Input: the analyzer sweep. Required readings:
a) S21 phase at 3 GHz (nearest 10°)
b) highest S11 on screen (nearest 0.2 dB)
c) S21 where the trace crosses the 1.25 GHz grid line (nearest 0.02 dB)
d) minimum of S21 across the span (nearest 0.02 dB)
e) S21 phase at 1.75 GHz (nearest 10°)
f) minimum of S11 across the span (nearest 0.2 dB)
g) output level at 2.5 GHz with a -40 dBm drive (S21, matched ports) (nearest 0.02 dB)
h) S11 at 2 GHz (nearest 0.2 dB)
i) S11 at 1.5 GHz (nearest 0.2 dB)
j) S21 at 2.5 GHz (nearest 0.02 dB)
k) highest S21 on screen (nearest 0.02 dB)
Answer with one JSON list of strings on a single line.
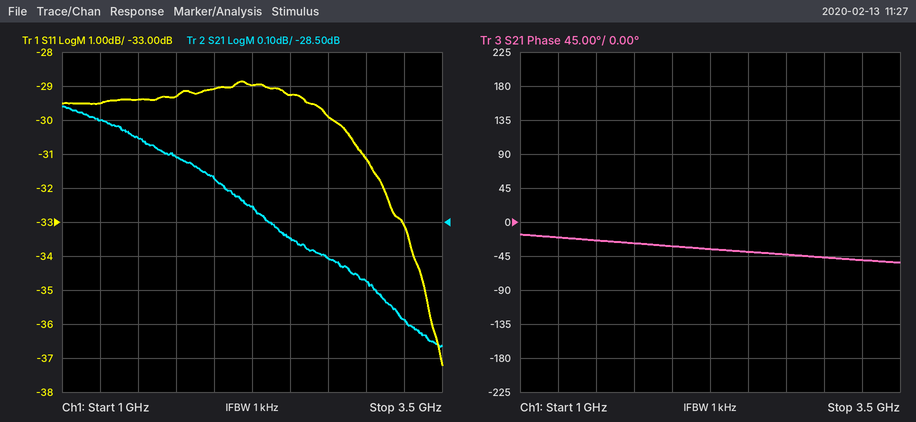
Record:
["-50°", "-28.8 dB", "-28.20 dB", "-28.86 dB", "-30°", "-37.2 dB", "-68.54 dBm", "-29.0 dB", "-29.4 dB", "-28.54 dB", "-28.16 dB"]
